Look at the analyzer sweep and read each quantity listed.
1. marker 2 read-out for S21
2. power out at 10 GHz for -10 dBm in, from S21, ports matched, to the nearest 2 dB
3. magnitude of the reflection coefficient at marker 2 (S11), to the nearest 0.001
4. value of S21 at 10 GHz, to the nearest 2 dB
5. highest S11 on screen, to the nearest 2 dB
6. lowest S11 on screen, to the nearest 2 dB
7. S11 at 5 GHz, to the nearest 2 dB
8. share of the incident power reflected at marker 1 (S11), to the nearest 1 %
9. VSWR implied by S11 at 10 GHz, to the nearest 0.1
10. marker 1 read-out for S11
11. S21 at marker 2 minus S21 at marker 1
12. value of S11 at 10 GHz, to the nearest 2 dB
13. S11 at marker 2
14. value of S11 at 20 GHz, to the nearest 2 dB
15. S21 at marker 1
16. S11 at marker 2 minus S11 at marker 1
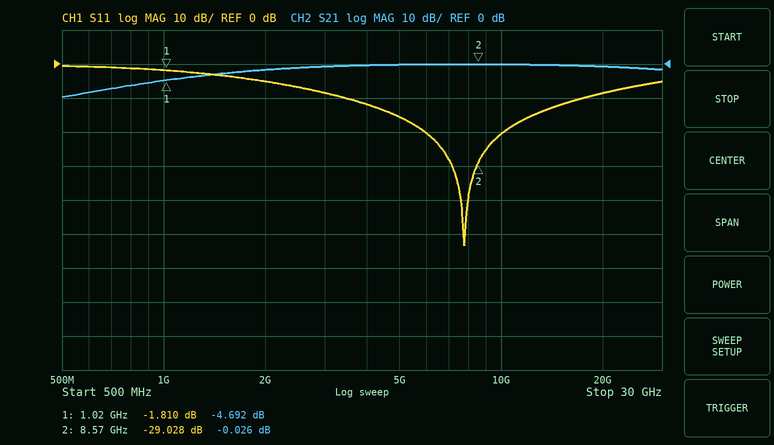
-0.026 dB
-10 dBm
0.035
0 dB
0 dB
-54 dB
-16 dB
66 %
1.2
-1.810 dB
4.666 dB
-20 dB
-29.028 dB
-8 dB
-4.692 dB
-27.218 dB
